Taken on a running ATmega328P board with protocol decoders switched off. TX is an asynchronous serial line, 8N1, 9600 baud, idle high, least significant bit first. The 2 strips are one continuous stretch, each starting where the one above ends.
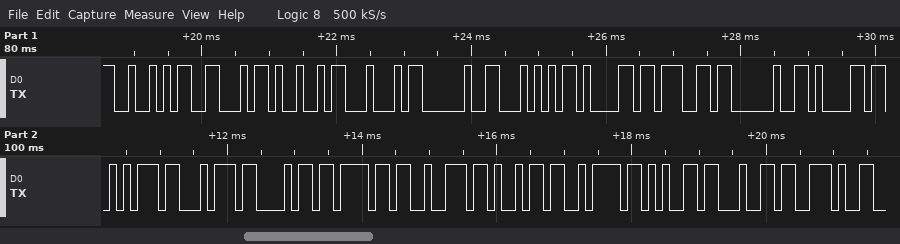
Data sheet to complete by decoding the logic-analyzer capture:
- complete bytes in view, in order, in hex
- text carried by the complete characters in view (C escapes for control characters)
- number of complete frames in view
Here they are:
52 46 49 44 20 54 61 67 20 61 75 74 68 6F 72 69 7A 65 64 2E
"RFID Tag authorized."
20
